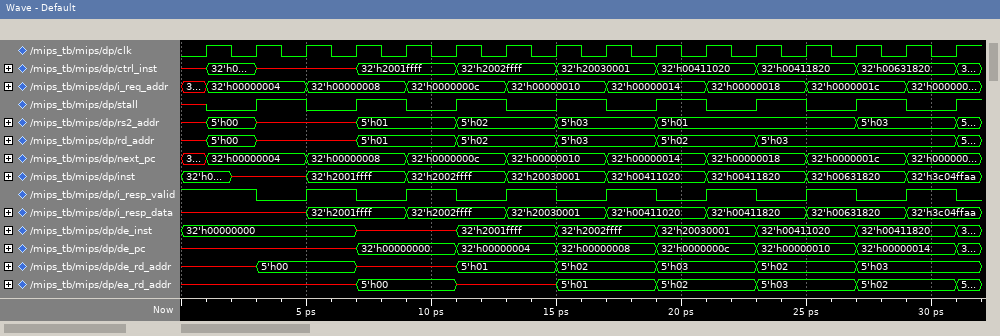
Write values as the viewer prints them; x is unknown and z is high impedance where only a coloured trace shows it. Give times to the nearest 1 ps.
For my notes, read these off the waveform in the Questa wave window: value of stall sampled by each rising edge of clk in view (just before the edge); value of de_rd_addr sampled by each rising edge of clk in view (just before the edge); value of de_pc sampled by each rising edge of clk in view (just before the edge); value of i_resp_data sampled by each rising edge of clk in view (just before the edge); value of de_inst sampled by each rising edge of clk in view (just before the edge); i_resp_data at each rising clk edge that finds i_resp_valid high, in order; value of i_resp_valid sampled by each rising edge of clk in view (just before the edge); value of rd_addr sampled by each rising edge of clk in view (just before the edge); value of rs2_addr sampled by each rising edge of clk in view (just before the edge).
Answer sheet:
x 0 1 0 1 0 1 0 1 0 1 0 1 0 1 0
x, x, 5'h00, 5'h00, x, x, 5'h01, 5'h01, 5'h02, 5'h02, 5'h03, 5'h03, 5'h02, 5'h02, 5'h03, 5'h03
x, x, x, x, 32'h00000000, 32'h00000000, 32'h00000004, 32'h00000004, 32'h00000008, 32'h00000008, 32'h0000000c, 32'h0000000c, 32'h00000010, 32'h00000010, 32'h00000014, 32'h00000014
x, x, x, 32'h2001ffff, 32'h2001ffff, 32'h2002ffff, 32'h2002ffff, 32'h20030001, 32'h20030001, 32'h00411020, 32'h00411020, 32'h00411820, 32'h00411820, 32'h00631820, 32'h00631820, 32'h3c04ffaa
32'h00000000, 32'h00000000, 32'h00000000, 32'h00000000, x, x, 32'h2001ffff, 32'h2001ffff, 32'h2002ffff, 32'h2002ffff, 32'h20030001, 32'h20030001, 32'h00411020, 32'h00411020, 32'h00411820, 32'h00411820
x, x, 32'h2001ffff, 32'h2002ffff, 32'h20030001, 32'h00411020, 32'h00411820, 32'h00631820, 32'h3c04ffaa
1 1 0 1 0 1 0 1 0 1 0 1 0 1 0 1
x, 5'h00, x, x, 5'h01, 5'h01, 5'h02, 5'h02, 5'h03, 5'h03, 5'h02, 5'h02, 5'h03, 5'h03, 5'h03, 5'h03
x, 5'h00, x, x, 5'h01, 5'h01, 5'h02, 5'h02, 5'h03, 5'h03, 5'h01, 5'h01, 5'h01, 5'h01, 5'h03, 5'h03
